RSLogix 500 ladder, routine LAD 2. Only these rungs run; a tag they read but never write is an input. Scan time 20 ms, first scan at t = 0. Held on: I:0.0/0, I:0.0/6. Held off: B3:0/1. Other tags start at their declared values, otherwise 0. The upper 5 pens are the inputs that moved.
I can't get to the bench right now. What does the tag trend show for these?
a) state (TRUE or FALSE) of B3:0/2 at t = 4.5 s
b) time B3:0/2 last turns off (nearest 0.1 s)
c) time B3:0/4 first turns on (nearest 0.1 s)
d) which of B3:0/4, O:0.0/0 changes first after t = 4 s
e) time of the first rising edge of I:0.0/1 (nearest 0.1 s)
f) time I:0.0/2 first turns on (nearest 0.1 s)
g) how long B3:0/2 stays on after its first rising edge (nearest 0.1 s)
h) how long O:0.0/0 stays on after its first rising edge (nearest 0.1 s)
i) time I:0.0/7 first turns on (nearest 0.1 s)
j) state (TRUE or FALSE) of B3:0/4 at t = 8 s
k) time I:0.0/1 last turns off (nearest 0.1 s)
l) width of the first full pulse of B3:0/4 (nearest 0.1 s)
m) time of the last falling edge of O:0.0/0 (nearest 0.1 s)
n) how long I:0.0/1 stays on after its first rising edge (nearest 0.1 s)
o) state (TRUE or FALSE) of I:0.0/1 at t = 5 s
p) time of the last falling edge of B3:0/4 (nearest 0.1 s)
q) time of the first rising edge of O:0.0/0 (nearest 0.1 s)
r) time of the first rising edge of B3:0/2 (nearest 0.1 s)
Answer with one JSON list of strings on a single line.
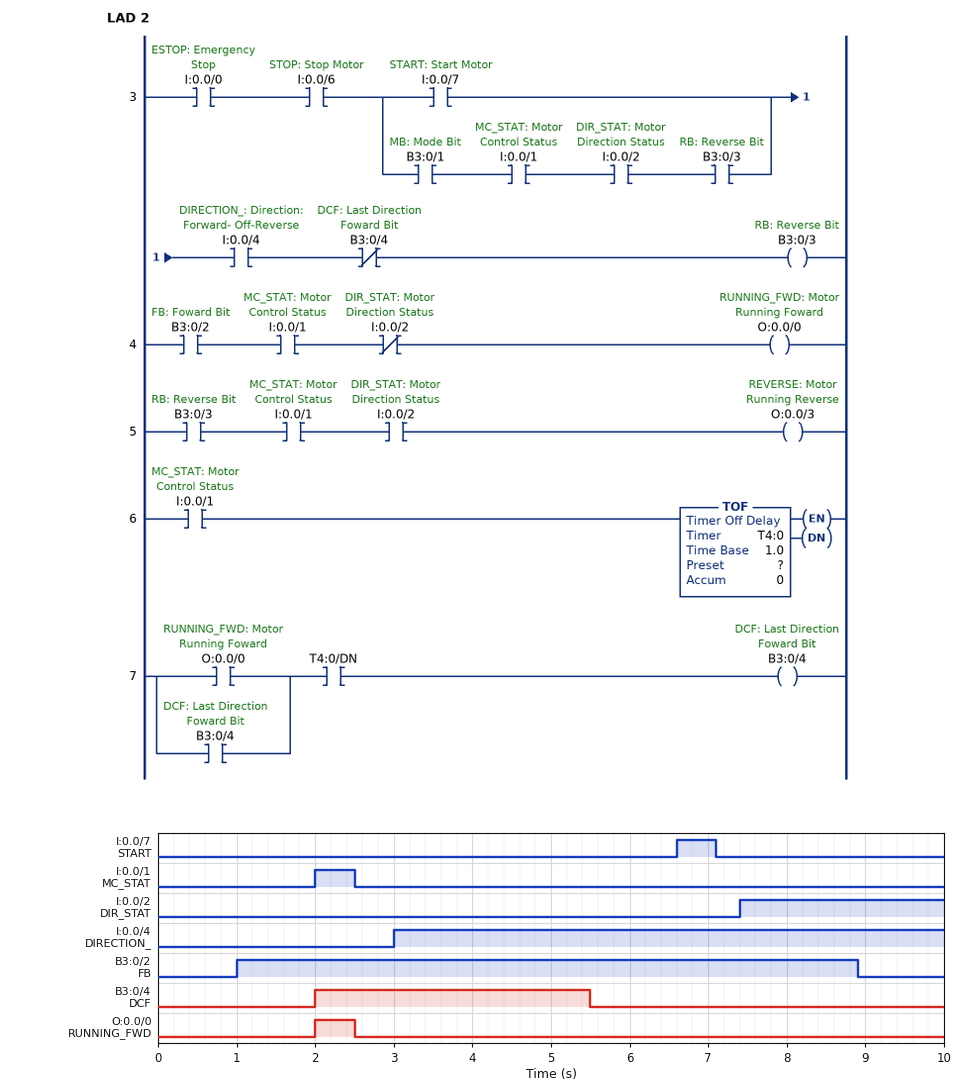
["TRUE", "8.9 s", "2.0 s", "B3:0/4", "2.0 s", "7.4 s", "7.9 s", "0.5 s", "6.6 s", "FALSE", "2.5 s", "3.5 s", "2.5 s", "0.5 s", "FALSE", "5.5 s", "2.0 s", "1.0 s"]
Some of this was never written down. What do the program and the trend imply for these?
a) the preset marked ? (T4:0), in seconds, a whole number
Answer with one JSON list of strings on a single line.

["3 s"]
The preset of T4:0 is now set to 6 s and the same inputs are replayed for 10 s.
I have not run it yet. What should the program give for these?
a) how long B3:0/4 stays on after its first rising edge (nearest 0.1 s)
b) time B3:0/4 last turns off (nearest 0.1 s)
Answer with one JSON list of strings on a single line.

["6.5 s", "8.5 s"]
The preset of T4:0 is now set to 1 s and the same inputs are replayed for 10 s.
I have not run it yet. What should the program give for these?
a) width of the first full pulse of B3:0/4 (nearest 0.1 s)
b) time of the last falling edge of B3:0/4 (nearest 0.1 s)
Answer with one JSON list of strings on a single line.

["1.5 s", "3.5 s"]
